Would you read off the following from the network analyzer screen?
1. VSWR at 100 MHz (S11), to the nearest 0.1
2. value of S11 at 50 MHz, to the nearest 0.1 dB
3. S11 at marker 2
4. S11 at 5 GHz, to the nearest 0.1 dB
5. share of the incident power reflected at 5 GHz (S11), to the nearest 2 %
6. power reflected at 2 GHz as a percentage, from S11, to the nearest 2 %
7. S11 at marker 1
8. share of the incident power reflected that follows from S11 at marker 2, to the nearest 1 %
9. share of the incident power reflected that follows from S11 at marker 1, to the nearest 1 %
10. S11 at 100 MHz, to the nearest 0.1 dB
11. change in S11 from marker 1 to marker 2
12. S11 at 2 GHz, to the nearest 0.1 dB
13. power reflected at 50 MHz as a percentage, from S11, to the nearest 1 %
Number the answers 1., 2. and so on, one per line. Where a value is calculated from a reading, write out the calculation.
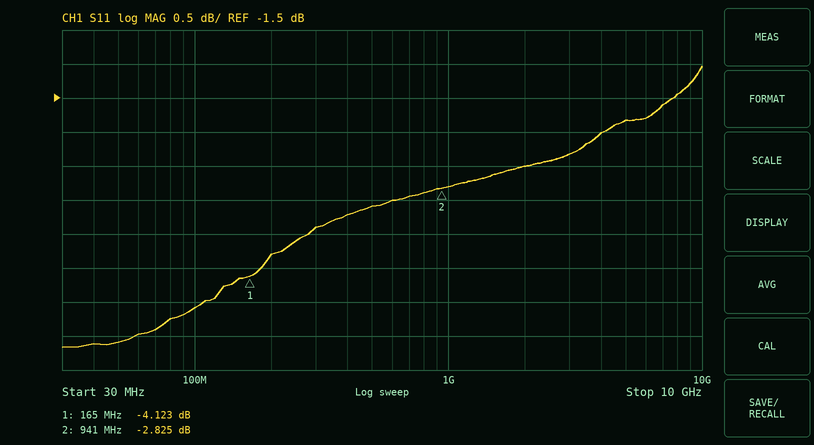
1. |Γ| = 10^(-4.6/20) = 0.5888; VSWR = (1 + 0.5888)/(1 − 0.5888) ≈ 3.9
2. -5.1 dB
3. -2.825 dB
4. -1.8 dB
5. 10^(-1.8/10) ≈ 66 %
6. 10^(-2.5/10) ≈ 56 %
7. -4.123 dB
8. 10^(-2.825/10) ≈ 52 %
9. 10^(-4.123/10) ≈ 39 %
10. -4.6 dB
11. -2.825 − (-4.123) = 1.298 dB
12. -2.5 dB
13. 10^(-5.1/10) ≈ 31 %
